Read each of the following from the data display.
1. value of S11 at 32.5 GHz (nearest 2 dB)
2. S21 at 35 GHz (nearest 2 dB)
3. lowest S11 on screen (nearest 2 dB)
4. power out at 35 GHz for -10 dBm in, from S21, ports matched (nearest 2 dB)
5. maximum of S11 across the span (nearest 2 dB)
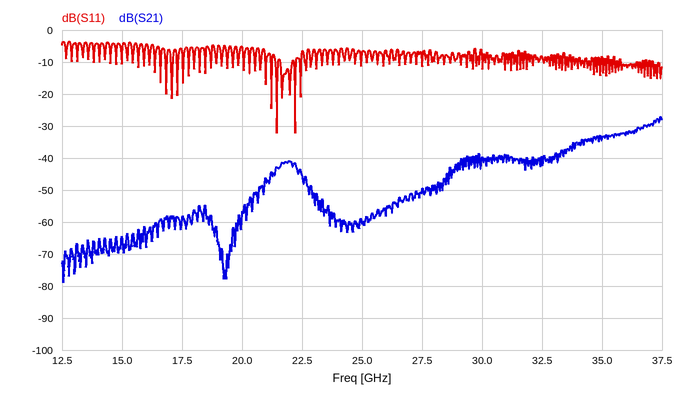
-8 dB
-34 dB
-32 dB
-44 dBm
-4 dB
